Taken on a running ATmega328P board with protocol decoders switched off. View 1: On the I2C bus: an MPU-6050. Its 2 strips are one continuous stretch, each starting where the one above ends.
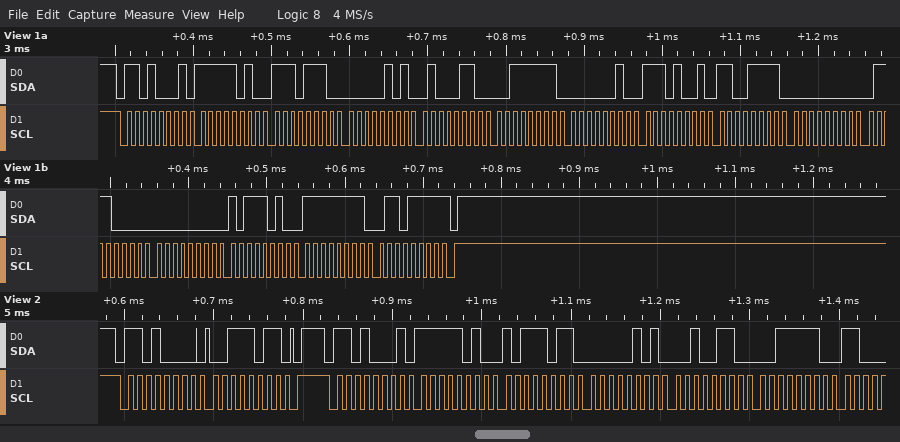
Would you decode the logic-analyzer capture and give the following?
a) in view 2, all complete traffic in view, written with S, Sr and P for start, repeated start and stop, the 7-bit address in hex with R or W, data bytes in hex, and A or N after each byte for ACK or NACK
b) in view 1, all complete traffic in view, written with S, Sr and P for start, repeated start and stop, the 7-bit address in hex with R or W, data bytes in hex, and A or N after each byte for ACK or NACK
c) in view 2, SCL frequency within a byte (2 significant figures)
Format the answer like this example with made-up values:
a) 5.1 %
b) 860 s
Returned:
a) S 68W A 3B A P S 68R A FA A BB A 05 A 26 A 3E A
b) S 68R A FA A EE A 05 A 46 A 3F A 02 A E9 A CF A 00 A 70 A 00 A BA A FF A 6F N P
c) 100 kHz
